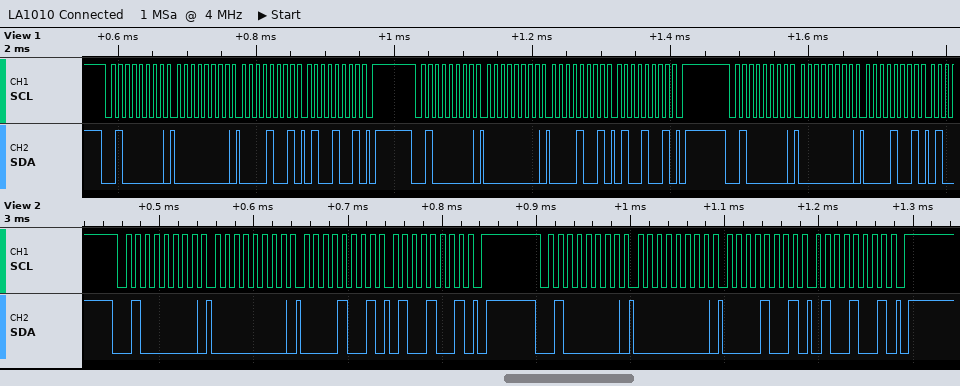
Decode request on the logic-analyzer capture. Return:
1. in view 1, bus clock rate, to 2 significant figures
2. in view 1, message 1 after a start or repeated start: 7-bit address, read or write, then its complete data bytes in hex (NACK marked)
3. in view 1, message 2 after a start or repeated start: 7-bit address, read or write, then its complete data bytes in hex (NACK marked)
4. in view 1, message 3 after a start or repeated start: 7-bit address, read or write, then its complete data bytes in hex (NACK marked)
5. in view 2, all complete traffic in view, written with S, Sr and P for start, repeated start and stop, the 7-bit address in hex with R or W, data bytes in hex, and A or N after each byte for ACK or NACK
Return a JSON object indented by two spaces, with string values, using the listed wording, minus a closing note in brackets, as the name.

{
  "in view 1, bus clock rate, to 2 significant figures": "100 kHz",
  "in view 1, message 1 after a start or repeated start: 7-bit address, read or write, then its complete data bytes in hex": "0x20 write: 00 09 49",
  "in view 1, message 2 after a start or repeated start: 7-bit address, read or write, then its complete data bytes in hex": "0x20 write: 00 09 49",
  "in view 1, message 3 after a start or repeated start: 7-bit address, read or write, then its complete data bytes in hex": "0x20 write: 00 09",
  "in view 2, all complete traffic in view, written with S, Sr and P for start, repeated start and stop, the 7-bit address in hex with R or W, data bytes in hex, and A or N after each byte for ACK or NACK": "S 20W A 00 A 09 A 49 A P S 20W A 00 A 09 A 49 A P"
}
